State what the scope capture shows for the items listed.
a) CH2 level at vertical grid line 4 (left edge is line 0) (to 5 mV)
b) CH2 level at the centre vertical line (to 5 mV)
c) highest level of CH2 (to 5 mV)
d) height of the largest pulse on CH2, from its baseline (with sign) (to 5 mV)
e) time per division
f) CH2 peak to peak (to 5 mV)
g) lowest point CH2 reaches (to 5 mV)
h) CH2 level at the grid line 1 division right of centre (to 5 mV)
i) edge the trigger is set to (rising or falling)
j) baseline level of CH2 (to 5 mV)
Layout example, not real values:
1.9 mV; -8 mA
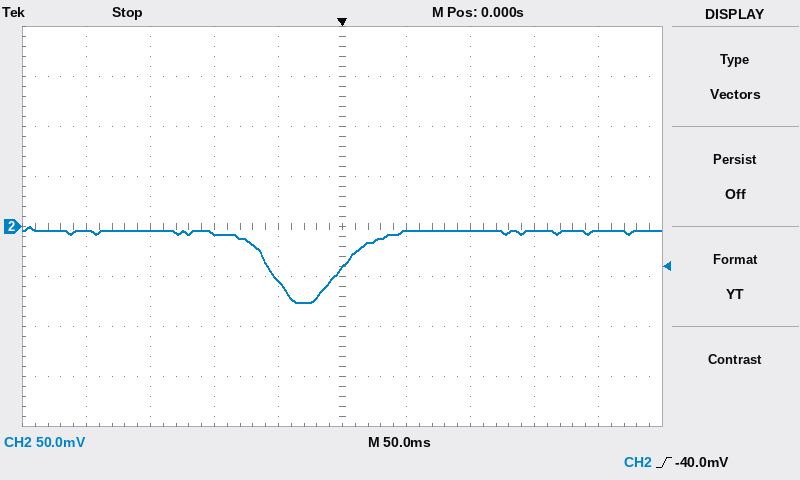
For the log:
-55 mV; -40 mV; 0 mV; -70 mV; 50 ms; 75 mV; -75 mV; -5 mV; rising; -5 mV
